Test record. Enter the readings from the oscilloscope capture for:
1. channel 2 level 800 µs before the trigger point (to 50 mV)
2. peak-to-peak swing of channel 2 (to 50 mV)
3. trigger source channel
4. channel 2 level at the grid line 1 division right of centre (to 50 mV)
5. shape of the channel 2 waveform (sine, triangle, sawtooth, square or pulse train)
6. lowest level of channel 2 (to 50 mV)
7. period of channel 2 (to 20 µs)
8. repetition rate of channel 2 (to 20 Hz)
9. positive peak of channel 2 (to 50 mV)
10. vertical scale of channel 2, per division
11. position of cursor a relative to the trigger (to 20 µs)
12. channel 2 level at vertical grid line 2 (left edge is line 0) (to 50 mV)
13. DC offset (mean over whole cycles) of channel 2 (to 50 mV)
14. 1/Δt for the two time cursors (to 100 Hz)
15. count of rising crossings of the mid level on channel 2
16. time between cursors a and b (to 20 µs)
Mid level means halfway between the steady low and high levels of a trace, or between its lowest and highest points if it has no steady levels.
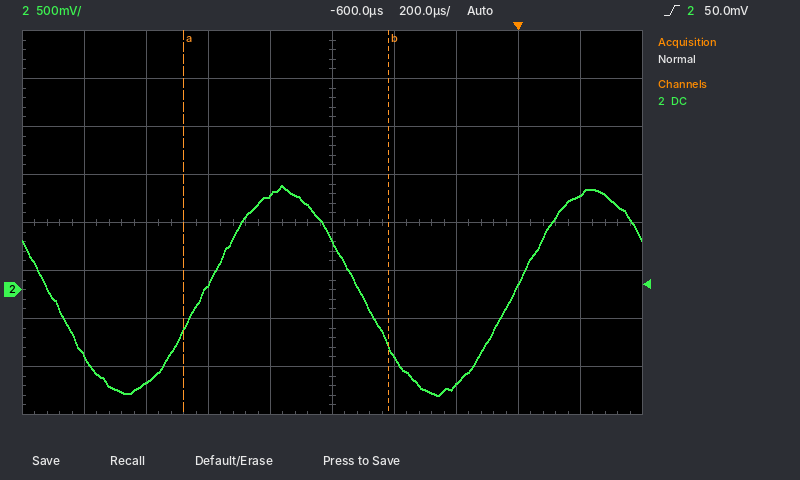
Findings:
1.00 V
2.20 V
channel 2
-700 mV
sine
-1.10 V
1.00 ms
1.00 kHz
1.10 V
500 mV
-1.08 ms
-950 mV
0 mV
1.5 kHz
2
660 µs
